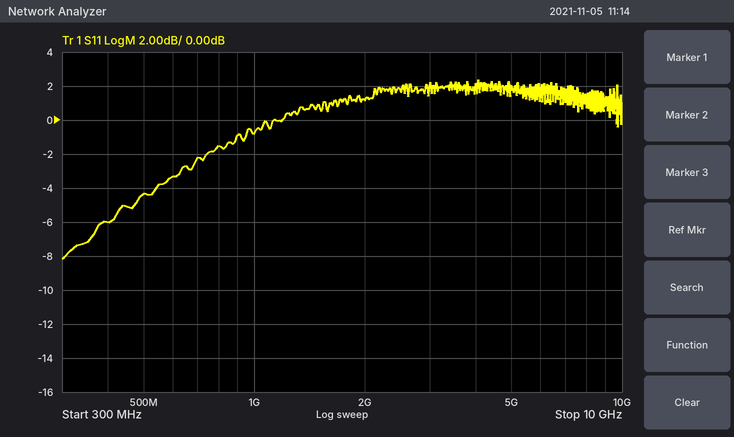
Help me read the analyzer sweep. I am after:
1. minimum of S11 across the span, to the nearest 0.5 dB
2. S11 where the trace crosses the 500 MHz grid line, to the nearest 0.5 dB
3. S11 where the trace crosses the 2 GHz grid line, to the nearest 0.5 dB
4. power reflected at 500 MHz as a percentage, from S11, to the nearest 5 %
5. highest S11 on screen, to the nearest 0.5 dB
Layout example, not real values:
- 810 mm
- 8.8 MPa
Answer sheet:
- -8.0 dB
- -4.5 dB
- 1.0 dB
- 35 %
- 2.5 dB
